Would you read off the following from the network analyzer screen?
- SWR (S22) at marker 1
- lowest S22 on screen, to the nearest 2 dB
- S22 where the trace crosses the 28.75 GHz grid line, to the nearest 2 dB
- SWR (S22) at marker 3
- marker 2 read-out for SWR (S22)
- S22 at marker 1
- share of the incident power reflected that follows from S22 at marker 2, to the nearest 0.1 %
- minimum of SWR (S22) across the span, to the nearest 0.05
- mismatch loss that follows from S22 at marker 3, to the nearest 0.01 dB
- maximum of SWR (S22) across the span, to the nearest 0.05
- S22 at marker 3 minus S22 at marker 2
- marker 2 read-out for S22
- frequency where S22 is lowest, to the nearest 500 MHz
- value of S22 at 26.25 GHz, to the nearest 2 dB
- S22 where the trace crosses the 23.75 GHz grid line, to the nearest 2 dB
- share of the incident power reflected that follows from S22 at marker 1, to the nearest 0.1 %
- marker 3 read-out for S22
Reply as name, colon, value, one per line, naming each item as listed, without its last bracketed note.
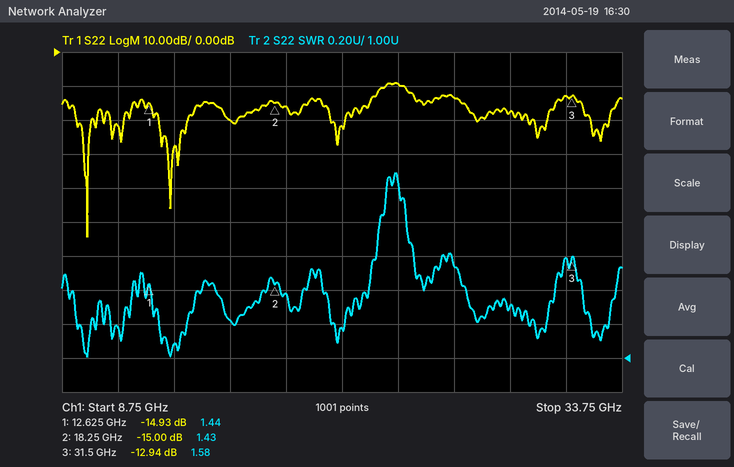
SWR (S22) at marker 1: 1.44
lowest S22 on screen, to the nearest 2 dB: -54 dB
S22 where the trace crosses the 28.75 GHz grid line, to the nearest 2 dB: -18 dB
SWR (S22) at marker 3: 1.58
marker 2 read-out for SWR: 1.43
S22 at marker 1: -14.93 dB
share of the incident power reflected that follows from S22 at marker 2, to the nearest 0.1 %: 3.2 %
minimum of SWR (S22) across the span, to the nearest 0.05: 1.00
mismatch loss that follows from S22 at marker 3, to the nearest 0.01 dB: 0.23 dB
maximum of SWR (S22) across the span, to the nearest 0.05: 2.10
S22 at marker 3 minus S22 at marker 2: 2.06 dB
marker 2 read-out for S22: -15.00 dB
frequency where S22 is lowest, to the nearest 500 MHz: 10.0 GHz
value of S22 at 26.25 GHz, to the nearest 2 dB: -14 dB
S22 where the trace crosses the 23.75 GHz grid line, to the nearest 2 dB: -10 dB
share of the incident power reflected that follows from S22 at marker 1, to the nearest 0.1 %: 3.2 %
marker 3 read-out for S22: -12.94 dB
